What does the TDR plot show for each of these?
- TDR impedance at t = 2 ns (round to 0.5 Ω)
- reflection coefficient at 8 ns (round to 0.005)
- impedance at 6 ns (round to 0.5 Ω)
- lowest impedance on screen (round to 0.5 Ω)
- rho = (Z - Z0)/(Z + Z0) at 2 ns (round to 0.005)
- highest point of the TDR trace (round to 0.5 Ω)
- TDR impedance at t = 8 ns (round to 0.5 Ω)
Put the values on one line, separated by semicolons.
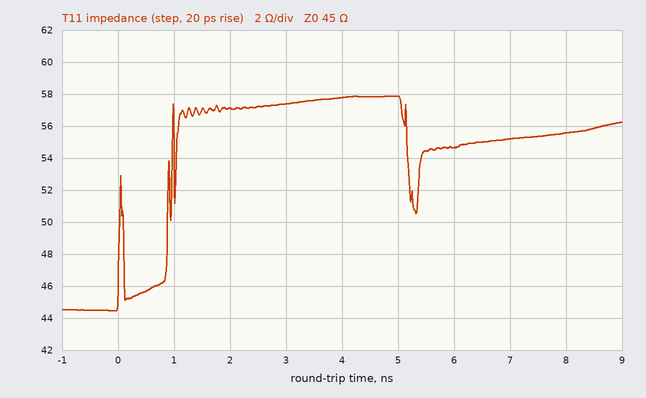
57.0 Ω; +0.105; 54.5 Ω; 44.5 Ω; +0.120; 58.0 Ω; 55.5 Ω
